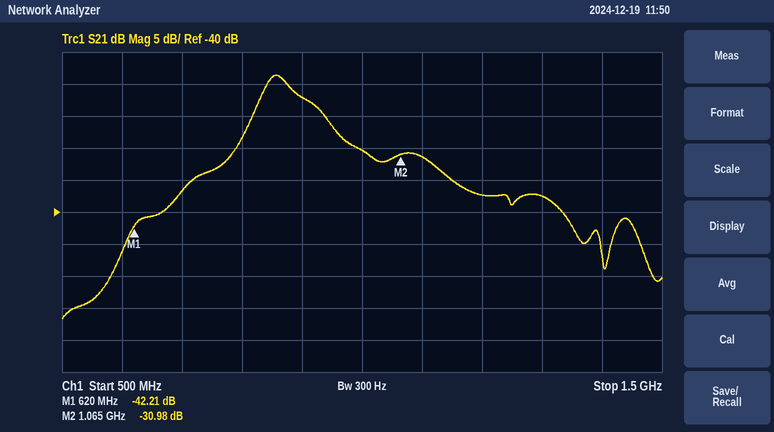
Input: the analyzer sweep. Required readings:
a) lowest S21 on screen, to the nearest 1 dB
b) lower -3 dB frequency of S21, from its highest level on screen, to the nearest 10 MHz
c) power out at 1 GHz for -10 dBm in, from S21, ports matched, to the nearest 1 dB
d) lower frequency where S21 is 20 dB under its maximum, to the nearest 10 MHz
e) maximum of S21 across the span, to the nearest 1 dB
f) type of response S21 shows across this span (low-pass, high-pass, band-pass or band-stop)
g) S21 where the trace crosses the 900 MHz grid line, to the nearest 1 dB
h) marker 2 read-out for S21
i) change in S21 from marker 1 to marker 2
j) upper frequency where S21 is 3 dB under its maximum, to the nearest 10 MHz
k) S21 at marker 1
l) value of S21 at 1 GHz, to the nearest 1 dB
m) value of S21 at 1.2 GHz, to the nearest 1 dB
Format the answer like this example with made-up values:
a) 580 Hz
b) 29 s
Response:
a) -57 dB
b) 830 MHz
c) -40 dBm
d) 680 MHz
e) -19 dB
f) band-pass
g) -22 dB
h) -30.98 dB
i) 11.23 dB
j) 890 MHz
k) -42.21 dB
l) -30 dB
m) -37 dB
